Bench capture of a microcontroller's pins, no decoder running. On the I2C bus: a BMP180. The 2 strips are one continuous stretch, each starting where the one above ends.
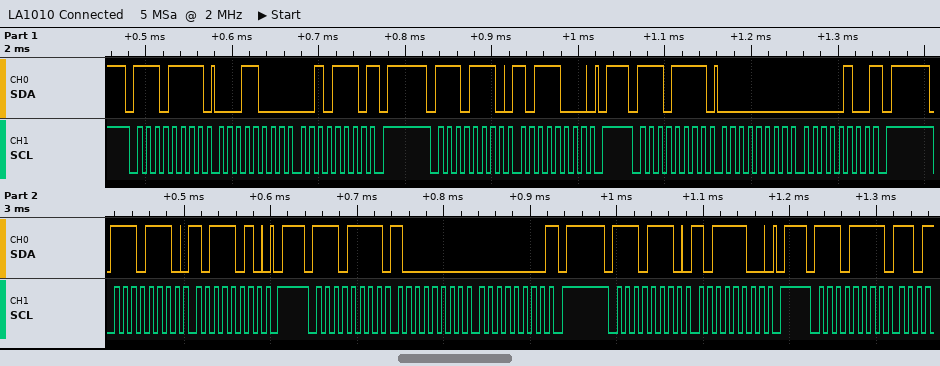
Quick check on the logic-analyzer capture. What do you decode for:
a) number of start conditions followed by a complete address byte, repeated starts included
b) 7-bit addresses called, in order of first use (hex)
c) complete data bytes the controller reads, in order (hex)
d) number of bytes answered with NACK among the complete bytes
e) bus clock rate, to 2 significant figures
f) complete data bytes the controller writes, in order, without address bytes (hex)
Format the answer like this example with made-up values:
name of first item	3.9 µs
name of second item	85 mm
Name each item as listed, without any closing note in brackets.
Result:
number of start conditions followed by a complete address byte, repeated starts included	7
7-bit addresses called, in order of first use	0x77
complete data bytes the controller reads, in order	18 2E 00 04 80 00
number of bytes answered with NACK among the complete bytes	3
bus clock rate, to 2 significant figures	100 kHz
complete data bytes the controller writes, in order, without address bytes	B8 BA BC
